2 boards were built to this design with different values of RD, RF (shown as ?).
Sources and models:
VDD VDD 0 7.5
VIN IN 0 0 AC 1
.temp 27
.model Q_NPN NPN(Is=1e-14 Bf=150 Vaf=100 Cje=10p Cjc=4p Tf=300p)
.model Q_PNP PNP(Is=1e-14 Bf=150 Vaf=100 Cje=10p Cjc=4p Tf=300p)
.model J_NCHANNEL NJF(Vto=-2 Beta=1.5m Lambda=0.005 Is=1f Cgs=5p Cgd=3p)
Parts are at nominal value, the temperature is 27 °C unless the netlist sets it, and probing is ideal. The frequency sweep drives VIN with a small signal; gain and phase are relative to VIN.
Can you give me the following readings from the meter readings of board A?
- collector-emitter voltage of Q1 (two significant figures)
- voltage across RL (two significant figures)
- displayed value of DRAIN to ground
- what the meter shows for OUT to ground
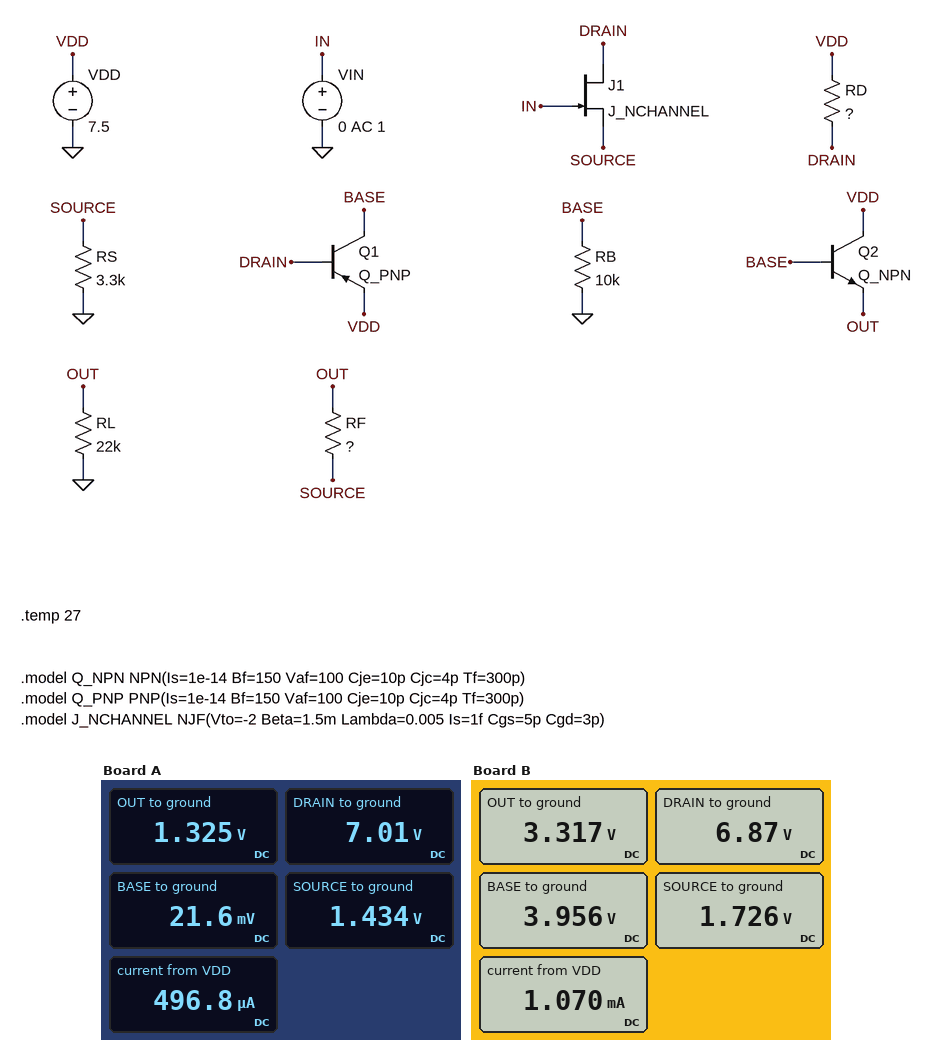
-7.5 V
1.3 V
7.01 V
1.325 V
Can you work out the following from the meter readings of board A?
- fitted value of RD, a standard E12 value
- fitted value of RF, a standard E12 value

1 kΩ
1.8 kΩ
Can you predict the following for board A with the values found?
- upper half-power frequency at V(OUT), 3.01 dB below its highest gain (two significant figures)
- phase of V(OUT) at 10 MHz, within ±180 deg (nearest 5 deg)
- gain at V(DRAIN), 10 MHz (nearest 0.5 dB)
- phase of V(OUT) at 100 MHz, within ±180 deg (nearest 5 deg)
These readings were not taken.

22 MHz
-20 deg
-12.5 dB
-50 deg
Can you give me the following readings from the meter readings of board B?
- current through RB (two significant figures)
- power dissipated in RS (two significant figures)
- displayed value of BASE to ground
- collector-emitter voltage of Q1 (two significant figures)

400 µA
900 µW
3.956 V
-3.5 V
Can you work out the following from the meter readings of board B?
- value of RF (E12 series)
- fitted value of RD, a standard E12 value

3.9 kΩ
5.6 kΩ
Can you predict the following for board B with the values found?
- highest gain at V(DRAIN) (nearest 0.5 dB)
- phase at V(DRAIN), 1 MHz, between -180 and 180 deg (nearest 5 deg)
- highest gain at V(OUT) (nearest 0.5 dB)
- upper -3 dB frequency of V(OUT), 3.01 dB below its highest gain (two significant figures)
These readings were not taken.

-24.5 dB
-170 deg
6.5 dB
15 MHz
